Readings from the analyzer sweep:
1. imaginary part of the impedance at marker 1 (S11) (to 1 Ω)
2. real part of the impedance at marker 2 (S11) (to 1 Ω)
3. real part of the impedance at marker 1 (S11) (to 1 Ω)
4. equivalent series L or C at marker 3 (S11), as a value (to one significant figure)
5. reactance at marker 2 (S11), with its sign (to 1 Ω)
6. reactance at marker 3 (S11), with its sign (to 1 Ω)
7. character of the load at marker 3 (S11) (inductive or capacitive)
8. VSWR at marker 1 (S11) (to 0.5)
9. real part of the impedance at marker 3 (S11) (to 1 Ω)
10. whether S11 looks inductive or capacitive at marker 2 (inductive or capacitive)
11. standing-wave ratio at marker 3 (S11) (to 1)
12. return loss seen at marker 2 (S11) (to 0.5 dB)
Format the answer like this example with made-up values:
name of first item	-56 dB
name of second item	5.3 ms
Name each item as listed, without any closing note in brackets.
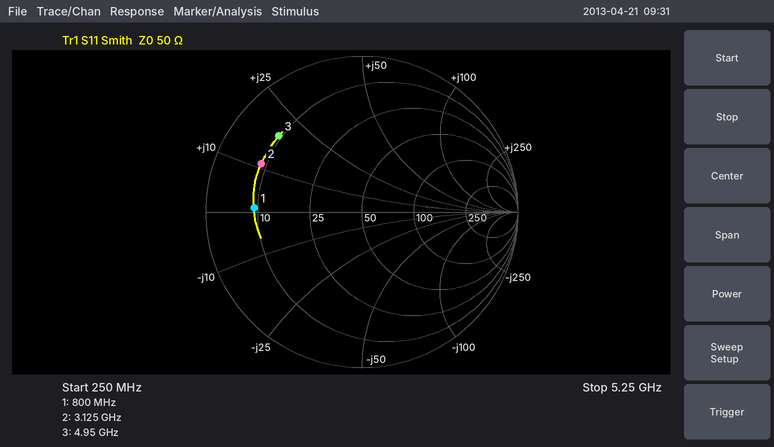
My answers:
imaginary part of the impedance at marker 1 (S11)	+1 Ω
real part of the impedance at marker 2 (S11)	9 Ω
real part of the impedance at marker 1 (S11)	9 Ω
equivalent series L or C at marker 3 (S11), as a value	600 pH
reactance at marker 2 (S11), with its sign	+11 Ω
reactance at marker 3 (S11), with its sign	+19 Ω
character of the load at marker 3 (S11)	inductive
VSWR at marker 1 (S11)	5.5
real part of the impedance at marker 3 (S11)	9 Ω
whether S11 looks inductive or capacitive at marker 2	inductive
standing-wave ratio at marker 3 (S11)	6
return loss seen at marker 2 (S11)	3.0 dB
